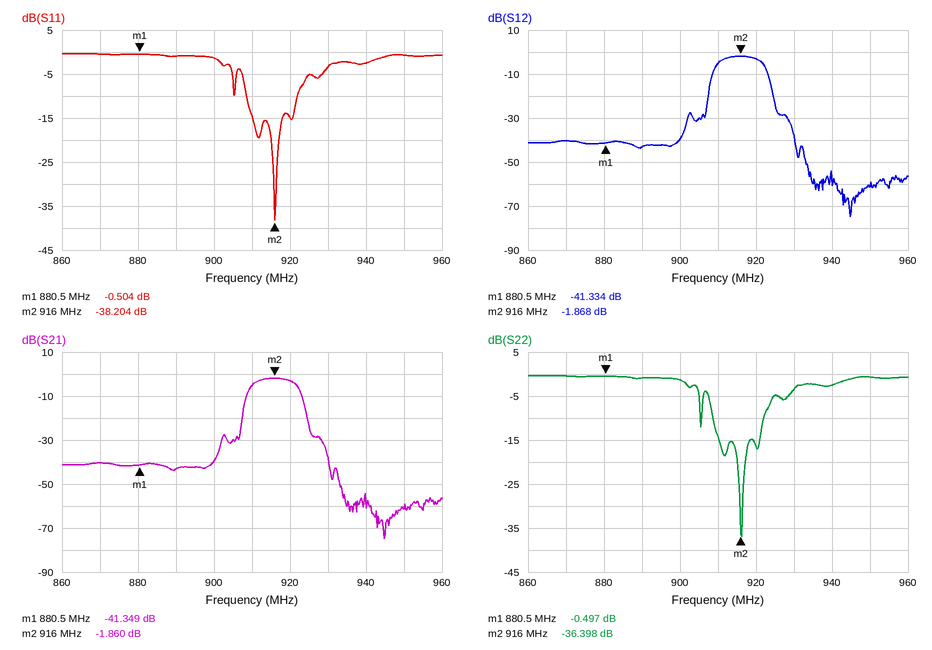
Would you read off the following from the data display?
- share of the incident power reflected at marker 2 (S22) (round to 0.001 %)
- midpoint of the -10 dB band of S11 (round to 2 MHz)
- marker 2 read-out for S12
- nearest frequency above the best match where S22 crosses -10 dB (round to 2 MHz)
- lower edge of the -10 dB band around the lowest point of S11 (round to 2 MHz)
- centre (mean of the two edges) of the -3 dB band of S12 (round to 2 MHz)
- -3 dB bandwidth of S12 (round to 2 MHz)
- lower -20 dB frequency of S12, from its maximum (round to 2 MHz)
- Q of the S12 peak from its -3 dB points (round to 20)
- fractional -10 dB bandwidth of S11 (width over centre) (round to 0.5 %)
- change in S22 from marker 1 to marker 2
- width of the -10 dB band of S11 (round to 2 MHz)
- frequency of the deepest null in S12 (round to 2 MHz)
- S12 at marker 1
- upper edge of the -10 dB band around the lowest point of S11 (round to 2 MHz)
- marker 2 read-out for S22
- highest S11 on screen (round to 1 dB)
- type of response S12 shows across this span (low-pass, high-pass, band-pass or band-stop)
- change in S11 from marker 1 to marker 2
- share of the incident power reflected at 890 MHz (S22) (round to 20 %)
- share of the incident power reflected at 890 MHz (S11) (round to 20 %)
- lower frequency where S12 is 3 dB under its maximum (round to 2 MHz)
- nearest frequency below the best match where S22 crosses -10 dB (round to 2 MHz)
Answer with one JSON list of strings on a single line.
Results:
["0.023 %", "916 MHz", "-1.868 dB", "922 MHz", "908 MHz", "916 MHz", "12 MHz", "908 MHz", "80", "1.5 %", "-35.901 dB", "14 MHz", "944 MHz", "-41.334 dB", "922 MHz", "-36.398 dB", "0 dB", "band-pass", "-37.700 dB", "80 %", "80 %", "910 MHz", "908 MHz"]
